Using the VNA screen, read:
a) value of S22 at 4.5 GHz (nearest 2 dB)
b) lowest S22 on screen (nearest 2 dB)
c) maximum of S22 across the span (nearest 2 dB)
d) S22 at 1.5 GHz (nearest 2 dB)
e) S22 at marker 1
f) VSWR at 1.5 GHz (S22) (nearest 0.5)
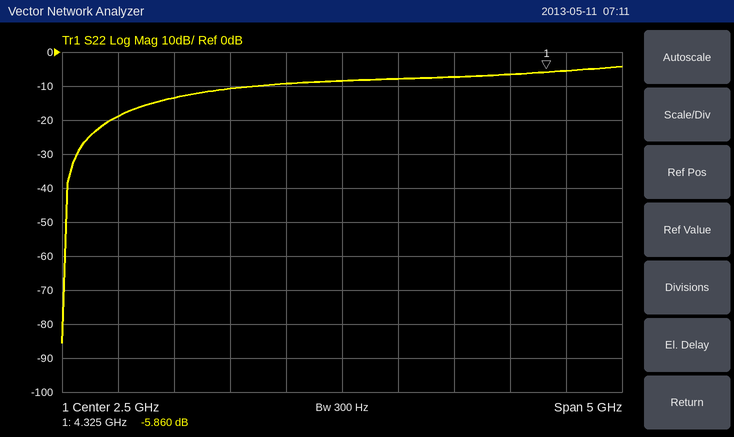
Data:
-6 dB
-86 dB
-4 dB
-10 dB
-5.860 dB
2.0
